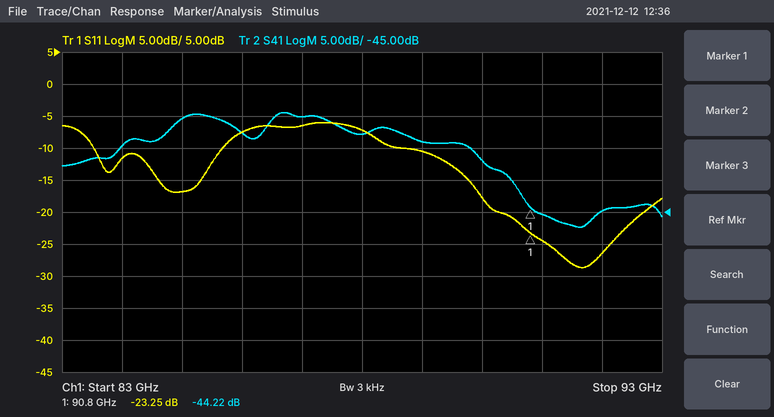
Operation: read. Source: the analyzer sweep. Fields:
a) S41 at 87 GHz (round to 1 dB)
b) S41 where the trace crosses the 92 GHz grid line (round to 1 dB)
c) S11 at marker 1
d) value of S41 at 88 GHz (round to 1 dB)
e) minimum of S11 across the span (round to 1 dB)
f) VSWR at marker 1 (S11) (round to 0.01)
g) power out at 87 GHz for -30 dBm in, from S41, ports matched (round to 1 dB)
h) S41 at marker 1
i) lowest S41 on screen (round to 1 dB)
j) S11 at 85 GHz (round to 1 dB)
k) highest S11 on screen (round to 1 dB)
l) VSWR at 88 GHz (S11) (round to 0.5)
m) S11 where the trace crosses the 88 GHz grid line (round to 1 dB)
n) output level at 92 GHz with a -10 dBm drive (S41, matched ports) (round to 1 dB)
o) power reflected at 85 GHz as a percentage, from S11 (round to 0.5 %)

-30 dB
-45 dB
-23.25 dB
-33 dB
-29 dB
1.15
-60 dBm
-44.22 dB
-47 dB
-17 dB
-6 dB
2.5
-7 dB
-55 dBm
2.0 %
